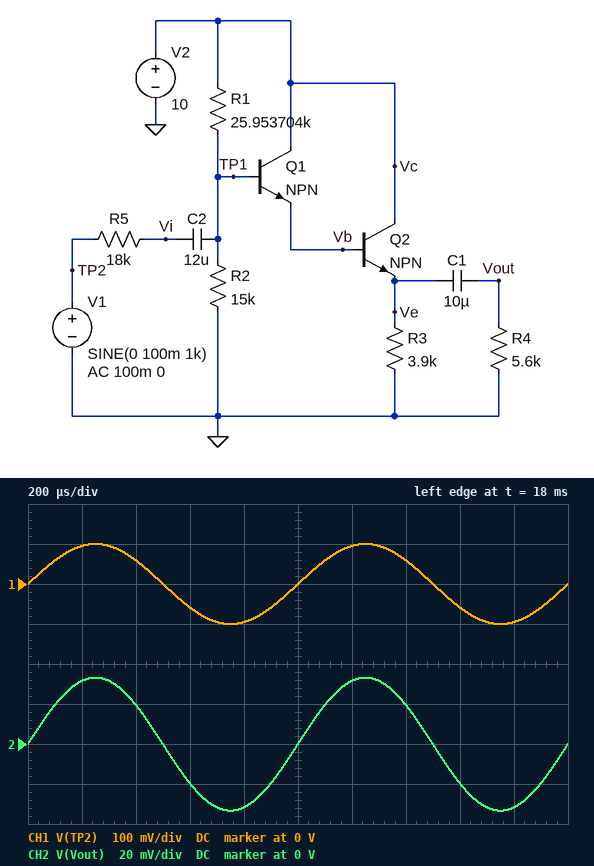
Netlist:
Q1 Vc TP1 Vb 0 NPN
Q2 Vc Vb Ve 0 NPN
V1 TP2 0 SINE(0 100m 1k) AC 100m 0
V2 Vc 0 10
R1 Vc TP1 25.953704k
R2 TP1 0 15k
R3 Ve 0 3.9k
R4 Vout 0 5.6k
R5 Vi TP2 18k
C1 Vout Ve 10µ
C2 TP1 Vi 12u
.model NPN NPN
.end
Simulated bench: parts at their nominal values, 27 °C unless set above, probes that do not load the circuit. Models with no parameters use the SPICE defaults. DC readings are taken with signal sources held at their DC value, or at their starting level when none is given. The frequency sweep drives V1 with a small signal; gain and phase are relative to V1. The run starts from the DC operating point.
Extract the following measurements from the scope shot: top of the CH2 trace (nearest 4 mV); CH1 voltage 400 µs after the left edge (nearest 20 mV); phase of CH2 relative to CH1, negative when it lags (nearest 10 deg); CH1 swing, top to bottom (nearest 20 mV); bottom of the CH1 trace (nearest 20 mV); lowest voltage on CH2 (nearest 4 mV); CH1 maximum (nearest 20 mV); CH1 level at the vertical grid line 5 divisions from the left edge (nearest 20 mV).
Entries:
32 mV
60 mV
0 deg
200 mV
-100 mV
-32 mV
100 mV
0 V
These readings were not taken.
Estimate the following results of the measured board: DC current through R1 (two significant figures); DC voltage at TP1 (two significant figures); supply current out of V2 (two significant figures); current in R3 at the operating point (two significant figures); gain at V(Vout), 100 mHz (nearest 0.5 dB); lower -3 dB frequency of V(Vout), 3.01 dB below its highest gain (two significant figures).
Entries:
240 µA
3.7 V
820 µA
580 µA
-52.5 dB
2.9 Hz
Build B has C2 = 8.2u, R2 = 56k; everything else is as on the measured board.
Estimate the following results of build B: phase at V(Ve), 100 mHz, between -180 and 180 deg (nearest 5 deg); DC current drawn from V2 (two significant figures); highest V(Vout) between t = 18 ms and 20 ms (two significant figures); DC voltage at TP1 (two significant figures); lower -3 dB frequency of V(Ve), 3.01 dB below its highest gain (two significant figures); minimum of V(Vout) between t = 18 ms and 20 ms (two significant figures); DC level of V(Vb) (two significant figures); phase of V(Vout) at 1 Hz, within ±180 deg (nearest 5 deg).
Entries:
80 deg
1.5 mA
49 mV
6.8 V
540 mHz
-49 mV
6.2 V
100 deg
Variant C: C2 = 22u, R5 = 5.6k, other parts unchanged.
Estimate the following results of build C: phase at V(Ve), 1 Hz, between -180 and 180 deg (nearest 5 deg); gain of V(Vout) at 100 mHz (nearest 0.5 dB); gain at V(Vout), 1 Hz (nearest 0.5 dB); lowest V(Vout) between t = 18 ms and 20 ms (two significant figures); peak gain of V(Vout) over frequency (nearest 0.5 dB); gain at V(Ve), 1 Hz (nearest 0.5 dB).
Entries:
25 deg
-47.0 dB
-14.5 dB
-61 mV
-4.5 dB
-5.0 dB
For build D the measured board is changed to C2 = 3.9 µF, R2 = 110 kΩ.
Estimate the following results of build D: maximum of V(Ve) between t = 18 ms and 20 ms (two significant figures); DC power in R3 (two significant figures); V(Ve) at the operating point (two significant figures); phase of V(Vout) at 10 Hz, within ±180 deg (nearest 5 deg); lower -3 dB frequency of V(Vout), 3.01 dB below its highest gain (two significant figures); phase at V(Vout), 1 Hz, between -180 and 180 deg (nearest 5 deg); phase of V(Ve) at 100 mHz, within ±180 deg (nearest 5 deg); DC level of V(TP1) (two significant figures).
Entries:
6.7 V
11 mW
6.6 V
20 deg
3.2 Hz
115 deg
85 deg
8.1 V
